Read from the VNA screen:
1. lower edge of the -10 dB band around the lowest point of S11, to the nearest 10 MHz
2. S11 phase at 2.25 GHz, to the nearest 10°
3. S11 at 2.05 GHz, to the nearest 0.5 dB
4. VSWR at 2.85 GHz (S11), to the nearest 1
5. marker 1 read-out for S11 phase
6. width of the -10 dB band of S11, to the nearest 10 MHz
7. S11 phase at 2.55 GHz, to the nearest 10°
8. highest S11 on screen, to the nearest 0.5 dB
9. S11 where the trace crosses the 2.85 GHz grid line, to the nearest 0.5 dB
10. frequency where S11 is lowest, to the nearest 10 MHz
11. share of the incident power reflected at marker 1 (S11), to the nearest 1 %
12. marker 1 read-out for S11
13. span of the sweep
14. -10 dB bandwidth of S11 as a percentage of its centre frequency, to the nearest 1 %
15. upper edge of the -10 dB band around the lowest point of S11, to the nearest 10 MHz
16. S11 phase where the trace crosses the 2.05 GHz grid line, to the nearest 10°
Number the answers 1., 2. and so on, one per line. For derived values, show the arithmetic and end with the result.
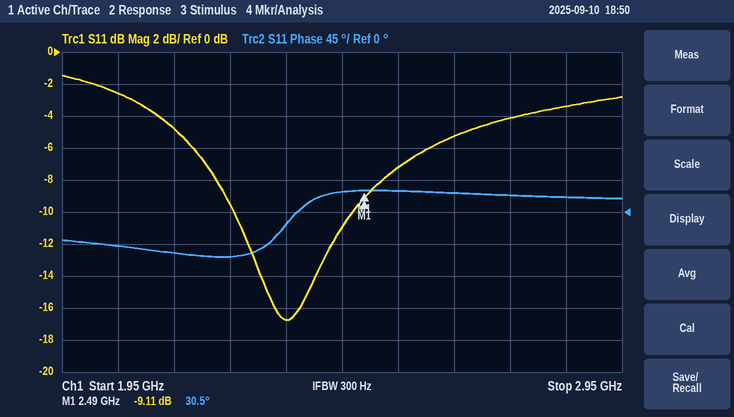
1. 2.26 GHz
2. -60°
3. -2.5 dB
4. |Γ| = 10^(-3.5/20) = 0.6683; VSWR = (1 + 0.6683)/(1 − 0.6683) ≈ 5
5. 30.5°
6. 2.47 GHz − 2.26 GHz = 210 MHz
7. 30°
8. -1.5 dB
9. -3.5 dB
10. 2.35 GHz
11. 10^(-9.11/10) ≈ 12 %
12. -9.11 dB
13. 1 GHz
14. 210 MHz / 2.365 GHz ≈ 9 %
15. 2.47 GHz
16. -50°
